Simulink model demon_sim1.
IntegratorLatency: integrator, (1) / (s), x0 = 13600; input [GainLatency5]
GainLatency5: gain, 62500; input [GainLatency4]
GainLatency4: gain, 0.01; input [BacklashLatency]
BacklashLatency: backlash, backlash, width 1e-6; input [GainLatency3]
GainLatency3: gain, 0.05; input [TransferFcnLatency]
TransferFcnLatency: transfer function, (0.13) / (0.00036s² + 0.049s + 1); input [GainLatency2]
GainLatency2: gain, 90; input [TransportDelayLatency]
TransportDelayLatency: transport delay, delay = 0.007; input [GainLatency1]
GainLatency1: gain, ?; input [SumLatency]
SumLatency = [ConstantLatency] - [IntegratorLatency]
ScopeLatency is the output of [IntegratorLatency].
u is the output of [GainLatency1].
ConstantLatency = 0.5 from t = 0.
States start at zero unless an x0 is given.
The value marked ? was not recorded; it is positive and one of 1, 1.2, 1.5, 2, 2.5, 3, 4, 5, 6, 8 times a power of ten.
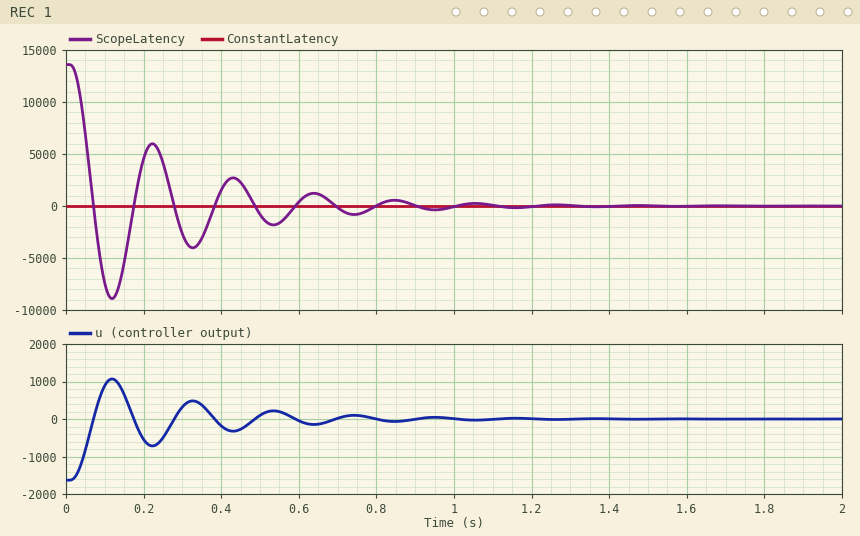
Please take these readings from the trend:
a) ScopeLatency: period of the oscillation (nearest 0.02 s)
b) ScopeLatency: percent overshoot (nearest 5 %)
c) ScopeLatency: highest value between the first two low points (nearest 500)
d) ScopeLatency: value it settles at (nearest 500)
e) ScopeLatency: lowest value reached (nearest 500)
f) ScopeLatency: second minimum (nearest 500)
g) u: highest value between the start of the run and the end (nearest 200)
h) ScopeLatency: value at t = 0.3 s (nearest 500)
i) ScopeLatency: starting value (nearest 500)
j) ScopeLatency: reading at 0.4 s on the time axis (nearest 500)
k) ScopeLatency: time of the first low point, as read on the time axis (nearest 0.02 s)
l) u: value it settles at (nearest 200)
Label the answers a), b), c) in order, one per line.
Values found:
a) 0.20 s
b) 65 %
c) 6000
d) 0
e) -9000
f) -4000
g) 1000
h) -2500
i) 13500
j) 1500
k) 0.12 s
l) 0
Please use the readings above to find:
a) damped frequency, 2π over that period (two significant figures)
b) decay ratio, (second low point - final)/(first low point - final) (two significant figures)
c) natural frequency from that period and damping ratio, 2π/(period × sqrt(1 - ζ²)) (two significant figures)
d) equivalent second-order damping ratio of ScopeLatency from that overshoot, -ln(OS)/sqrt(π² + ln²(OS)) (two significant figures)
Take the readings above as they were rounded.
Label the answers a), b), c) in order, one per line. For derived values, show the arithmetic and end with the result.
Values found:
a) 2π / 0.2 = 31 rad/s
b) (-4000 - 0) / (-9000 - 0) = 0.44
c) 2π / (0.2 × sqrt(1 - 0.14²)) = 32 rad/s
d) ln(0.65) = -0.431; 0.431 / sqrt(9.870 + 0.186) = 0.14
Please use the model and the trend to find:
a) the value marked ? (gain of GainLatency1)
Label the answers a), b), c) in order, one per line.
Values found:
a) 0.12
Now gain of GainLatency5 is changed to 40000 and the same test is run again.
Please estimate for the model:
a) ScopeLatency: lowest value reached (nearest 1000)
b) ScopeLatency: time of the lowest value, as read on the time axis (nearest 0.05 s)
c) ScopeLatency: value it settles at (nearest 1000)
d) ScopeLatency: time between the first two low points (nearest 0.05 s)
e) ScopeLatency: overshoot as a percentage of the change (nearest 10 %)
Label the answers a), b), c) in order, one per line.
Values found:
a) -6000
b) 0.15 s
c) 0
d) 0.25 s
e) 40 %
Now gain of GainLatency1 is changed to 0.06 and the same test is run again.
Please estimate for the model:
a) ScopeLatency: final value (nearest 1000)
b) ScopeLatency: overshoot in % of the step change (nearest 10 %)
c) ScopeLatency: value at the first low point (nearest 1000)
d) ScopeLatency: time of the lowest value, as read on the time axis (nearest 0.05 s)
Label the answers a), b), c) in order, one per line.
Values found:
a) 0
b) 30 %
c) -4000
d) 0.15 s
